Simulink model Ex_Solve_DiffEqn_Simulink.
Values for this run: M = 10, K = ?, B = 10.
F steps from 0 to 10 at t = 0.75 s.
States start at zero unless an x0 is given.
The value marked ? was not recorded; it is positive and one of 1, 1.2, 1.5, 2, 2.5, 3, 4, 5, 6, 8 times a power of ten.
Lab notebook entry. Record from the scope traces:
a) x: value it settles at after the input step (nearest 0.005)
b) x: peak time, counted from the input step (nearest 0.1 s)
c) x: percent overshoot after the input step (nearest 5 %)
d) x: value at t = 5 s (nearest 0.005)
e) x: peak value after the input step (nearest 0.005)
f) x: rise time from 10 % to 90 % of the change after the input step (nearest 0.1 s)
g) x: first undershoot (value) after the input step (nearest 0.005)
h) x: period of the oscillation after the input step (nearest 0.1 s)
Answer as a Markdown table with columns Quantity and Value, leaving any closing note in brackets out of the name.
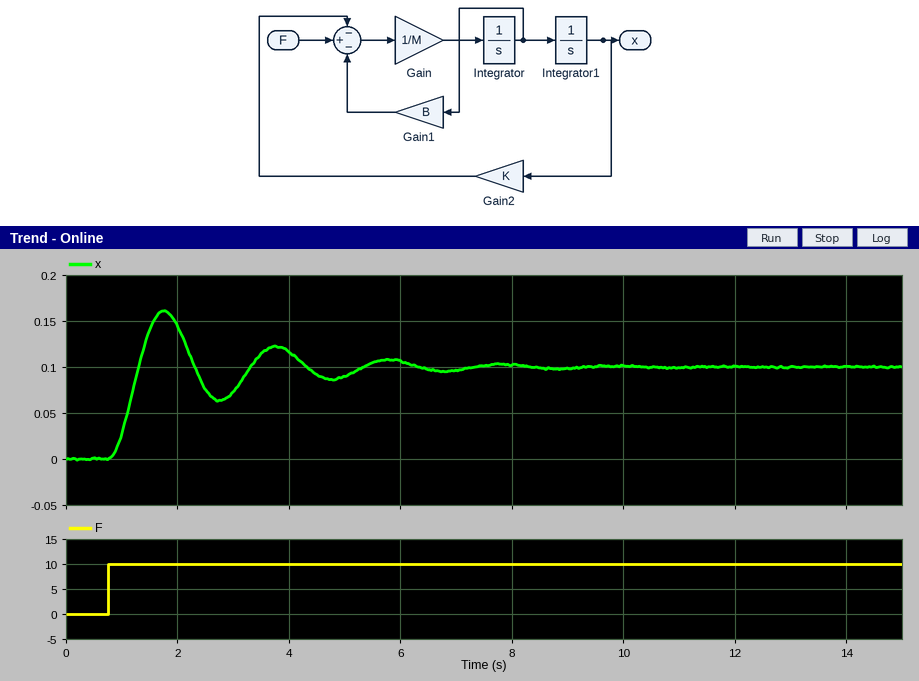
| Quantity | Value |
|---|---|
| x: value it settles at after the input step | 0.100 |
| x: peak time, counted from the input step | 1.0 s |
| x: percent overshoot after the input step | 60 % |
| x: value at t = 5 s | 0.090 |
| x: peak value after the input step | 0.160 |
| x: rise time from 10 % to 90 % of the change after the input step | 0.4 s |
| x: first undershoot (value) after the input step | 0.065 |
| x: period of the oscillation after the input step | 2.0 s |
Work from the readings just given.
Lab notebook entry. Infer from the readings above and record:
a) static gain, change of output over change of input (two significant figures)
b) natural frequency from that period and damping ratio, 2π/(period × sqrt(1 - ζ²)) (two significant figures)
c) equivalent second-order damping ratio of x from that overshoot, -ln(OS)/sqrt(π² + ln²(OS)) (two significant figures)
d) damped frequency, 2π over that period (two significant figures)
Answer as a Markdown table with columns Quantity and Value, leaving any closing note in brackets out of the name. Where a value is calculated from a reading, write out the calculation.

| Quantity | Value |
|---|---|
| static gain, change of output over change of input | (0.1 - 0) / (10 - 0) = 0.010 |
| natural frequency from that period and damping ratio, 2π/(period × sqrt(1 - ζ²)) | 2π / (2 × sqrt(1 - 0.16²)) = 3.2 rad/s |
| equivalent second-order damping ratio of x from that overshoot, -ln(OS)/sqrt(π² + ln²(OS)) | ln(0.6) = -0.511; 0.511 / sqrt(9.870 + 0.261) = 0.16 |
| damped frequency, 2π over that period | 2π / 2 = 3.1 rad/s |
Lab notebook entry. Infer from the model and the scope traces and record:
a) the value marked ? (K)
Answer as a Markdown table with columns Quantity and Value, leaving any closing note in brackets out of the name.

| Quantity | Value |
|---|---|
| the value marked ? | 100 |
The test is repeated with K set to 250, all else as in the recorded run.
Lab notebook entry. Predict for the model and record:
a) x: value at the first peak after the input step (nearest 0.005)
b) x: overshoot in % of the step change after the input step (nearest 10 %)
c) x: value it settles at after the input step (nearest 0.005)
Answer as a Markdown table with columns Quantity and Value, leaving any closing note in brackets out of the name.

| Quantity | Value |
|---|---|
| x: value at the first peak after the input step | 0.070 |
| x: overshoot in % of the step change after the input step | 70 % |
| x: value it settles at after the input step | 0.040 |
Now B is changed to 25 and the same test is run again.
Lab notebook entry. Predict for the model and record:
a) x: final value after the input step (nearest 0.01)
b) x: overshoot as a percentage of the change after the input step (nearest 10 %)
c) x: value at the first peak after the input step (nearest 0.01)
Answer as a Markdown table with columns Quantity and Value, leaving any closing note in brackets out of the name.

| Quantity | Value |
|---|---|
| x: final value after the input step | 0.10 |
| x: overshoot as a percentage of the change after the input step | 30 % |
| x: value at the first peak after the input step | 0.13 |
